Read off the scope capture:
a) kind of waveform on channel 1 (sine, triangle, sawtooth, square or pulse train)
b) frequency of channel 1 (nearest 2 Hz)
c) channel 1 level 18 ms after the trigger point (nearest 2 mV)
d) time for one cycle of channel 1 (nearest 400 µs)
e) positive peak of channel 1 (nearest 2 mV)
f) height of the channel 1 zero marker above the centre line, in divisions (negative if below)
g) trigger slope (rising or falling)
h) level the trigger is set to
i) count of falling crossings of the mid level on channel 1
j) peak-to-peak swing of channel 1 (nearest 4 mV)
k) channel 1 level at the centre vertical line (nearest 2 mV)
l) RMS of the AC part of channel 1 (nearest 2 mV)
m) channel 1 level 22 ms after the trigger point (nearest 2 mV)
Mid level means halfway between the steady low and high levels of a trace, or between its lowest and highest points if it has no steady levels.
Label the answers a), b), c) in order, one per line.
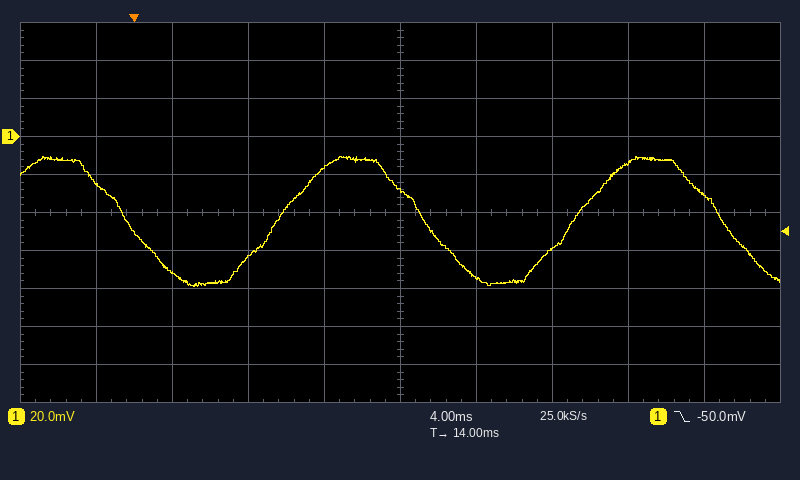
a) sine
b) 64 Hz
c) -74 mV
d) 15.6 ms
e) -10 mV
f) +2.0 div
g) falling
h) -50.0 mV
i) 3
j) 68 mV
k) -28 mV
l) 24 mV
m) -58 mV
